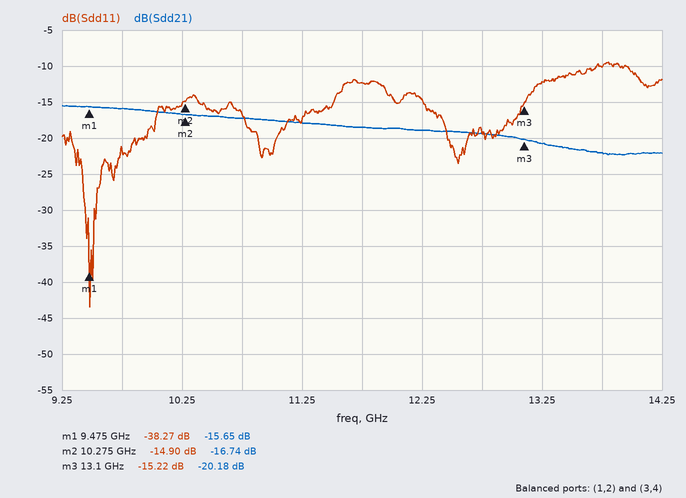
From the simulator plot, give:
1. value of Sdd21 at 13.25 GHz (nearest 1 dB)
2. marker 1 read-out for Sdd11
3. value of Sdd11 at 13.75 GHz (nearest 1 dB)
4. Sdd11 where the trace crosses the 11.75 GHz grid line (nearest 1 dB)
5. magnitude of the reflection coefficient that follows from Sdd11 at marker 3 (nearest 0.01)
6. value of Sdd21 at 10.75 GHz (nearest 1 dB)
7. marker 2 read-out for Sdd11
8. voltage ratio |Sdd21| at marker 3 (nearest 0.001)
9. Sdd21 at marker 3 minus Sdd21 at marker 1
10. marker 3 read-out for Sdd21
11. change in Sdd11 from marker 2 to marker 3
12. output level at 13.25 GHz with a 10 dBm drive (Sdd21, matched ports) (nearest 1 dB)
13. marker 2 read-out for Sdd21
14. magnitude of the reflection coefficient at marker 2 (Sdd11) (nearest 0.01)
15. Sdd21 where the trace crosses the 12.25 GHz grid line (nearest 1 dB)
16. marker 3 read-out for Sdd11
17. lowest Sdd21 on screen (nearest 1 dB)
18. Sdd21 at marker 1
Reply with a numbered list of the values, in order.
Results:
1. -21 dB
2. -38.27 dB
3. -10 dB
4. -12 dB
5. 0.17
6. -17 dB
7. -14.90 dB
8. 0.098
9. -4.53 dB
10. -20.18 dB
11. -0.32 dB
12. -11 dBm
13. -16.74 dB
14. 0.18
15. -19 dB
16. -15.22 dB
17. -22 dB
18. -15.65 dB
